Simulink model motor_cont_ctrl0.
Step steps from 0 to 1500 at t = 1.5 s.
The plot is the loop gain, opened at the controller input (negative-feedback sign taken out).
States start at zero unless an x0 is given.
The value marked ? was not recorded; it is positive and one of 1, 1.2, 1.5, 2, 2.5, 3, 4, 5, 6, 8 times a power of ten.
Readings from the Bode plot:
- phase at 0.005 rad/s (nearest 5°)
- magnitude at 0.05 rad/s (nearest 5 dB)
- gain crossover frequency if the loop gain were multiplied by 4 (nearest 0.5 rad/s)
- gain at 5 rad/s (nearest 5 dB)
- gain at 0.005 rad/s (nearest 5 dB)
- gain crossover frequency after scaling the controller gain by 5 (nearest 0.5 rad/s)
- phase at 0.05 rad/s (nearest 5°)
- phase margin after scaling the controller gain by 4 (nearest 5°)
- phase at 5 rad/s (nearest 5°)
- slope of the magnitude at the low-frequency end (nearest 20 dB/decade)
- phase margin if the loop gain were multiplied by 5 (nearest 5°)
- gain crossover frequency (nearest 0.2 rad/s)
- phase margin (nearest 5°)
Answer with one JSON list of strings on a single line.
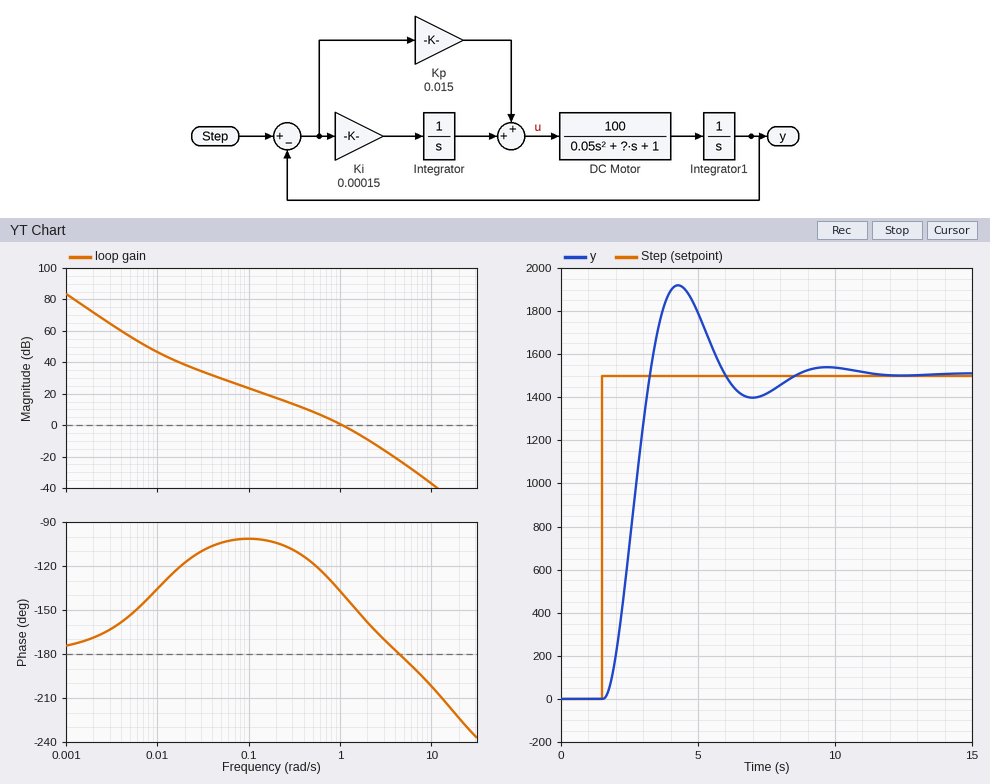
["-155°", "30 dB", "2.5 rad/s", "-25 dB", "55 dB", "2.5 rad/s", "-105°", "15°", "-185°", "-40 dB/decade", "15°", "1.0 rad/s", "40°"]
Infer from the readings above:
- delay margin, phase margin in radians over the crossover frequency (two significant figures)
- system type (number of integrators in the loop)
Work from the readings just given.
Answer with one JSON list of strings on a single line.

["0.70 s", "2"]
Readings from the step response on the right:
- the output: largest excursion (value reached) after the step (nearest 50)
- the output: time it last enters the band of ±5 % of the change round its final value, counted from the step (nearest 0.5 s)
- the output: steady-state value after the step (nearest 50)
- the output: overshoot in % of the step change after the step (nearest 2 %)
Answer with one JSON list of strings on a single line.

["1900", "6.0 s", "1500", "28 %"]
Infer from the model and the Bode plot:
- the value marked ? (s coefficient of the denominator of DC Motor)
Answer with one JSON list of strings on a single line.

["1"]
